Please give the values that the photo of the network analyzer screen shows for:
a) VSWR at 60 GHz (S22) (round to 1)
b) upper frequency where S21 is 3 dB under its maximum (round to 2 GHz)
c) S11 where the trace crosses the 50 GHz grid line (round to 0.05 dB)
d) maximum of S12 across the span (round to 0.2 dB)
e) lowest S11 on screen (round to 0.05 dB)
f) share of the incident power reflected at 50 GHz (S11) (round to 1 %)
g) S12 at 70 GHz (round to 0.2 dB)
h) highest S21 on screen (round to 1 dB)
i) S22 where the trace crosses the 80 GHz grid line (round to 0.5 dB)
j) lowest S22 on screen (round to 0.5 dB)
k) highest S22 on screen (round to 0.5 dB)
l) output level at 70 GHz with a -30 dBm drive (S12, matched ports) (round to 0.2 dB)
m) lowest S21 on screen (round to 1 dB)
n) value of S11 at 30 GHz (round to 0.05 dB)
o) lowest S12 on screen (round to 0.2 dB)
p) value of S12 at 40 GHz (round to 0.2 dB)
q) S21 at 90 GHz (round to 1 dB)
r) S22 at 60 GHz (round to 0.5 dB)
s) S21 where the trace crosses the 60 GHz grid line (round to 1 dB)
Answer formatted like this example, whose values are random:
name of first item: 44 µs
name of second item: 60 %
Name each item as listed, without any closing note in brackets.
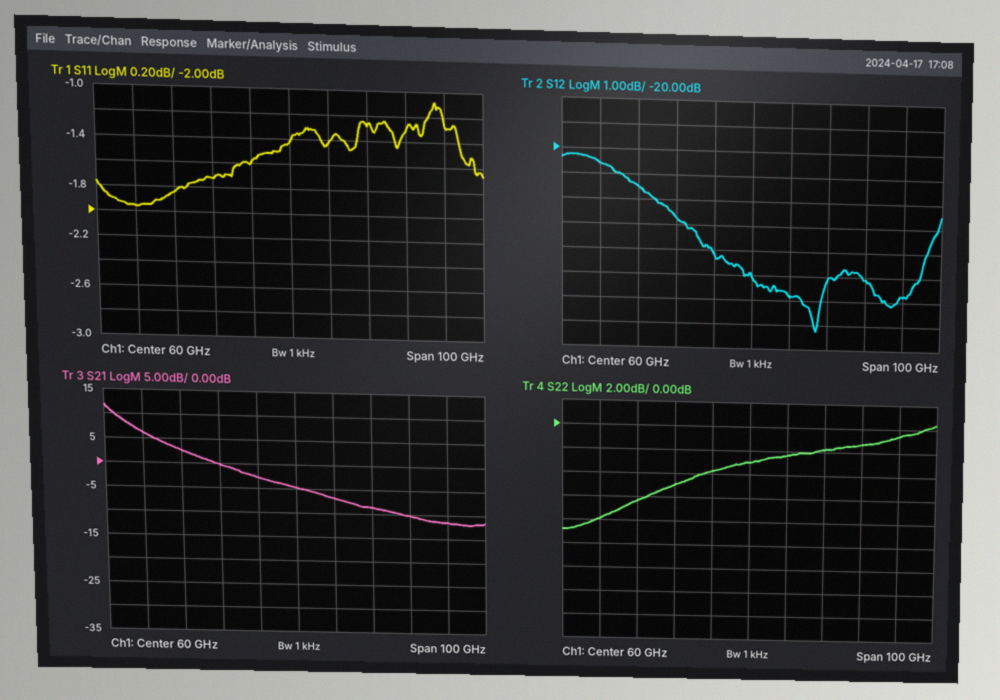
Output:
VSWR at 60 GHz (S22): 6
upper frequency where S21 is 3 dB under its maximum: 14 GHz
S11 where the trace crosses the 50 GHz grid line: -1.60 dB
maximum of S12 across the span: -20.2 dB
lowest S11 on screen: -1.95 dB
share of the incident power reflected at 50 GHz (S11): 69 %
S12 at 70 GHz: -25.8 dB
highest S21 on screen: 12 dB
S22 where the trace crosses the 80 GHz grid line: -2.0 dB
lowest S22 on screen: -9.0 dB
highest S22 on screen: 0.5 dB
output level at 70 GHz with a -30 dBm drive (S12, matched ports): -55.8 dBm
lowest S21 on screen: -12 dB
value of S11 at 30 GHz: -1.85 dB
lowest S12 on screen: -27.2 dB
value of S12 at 40 GHz: -22.8 dB
S21 at 90 GHz: -10 dB
S22 at 60 GHz: -3.0 dB
S21 where the trace crosses the 60 GHz grid line: -5 dB
